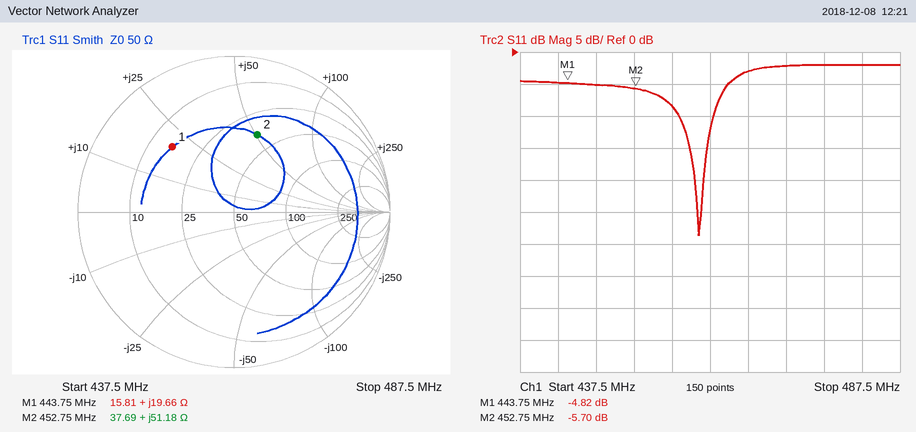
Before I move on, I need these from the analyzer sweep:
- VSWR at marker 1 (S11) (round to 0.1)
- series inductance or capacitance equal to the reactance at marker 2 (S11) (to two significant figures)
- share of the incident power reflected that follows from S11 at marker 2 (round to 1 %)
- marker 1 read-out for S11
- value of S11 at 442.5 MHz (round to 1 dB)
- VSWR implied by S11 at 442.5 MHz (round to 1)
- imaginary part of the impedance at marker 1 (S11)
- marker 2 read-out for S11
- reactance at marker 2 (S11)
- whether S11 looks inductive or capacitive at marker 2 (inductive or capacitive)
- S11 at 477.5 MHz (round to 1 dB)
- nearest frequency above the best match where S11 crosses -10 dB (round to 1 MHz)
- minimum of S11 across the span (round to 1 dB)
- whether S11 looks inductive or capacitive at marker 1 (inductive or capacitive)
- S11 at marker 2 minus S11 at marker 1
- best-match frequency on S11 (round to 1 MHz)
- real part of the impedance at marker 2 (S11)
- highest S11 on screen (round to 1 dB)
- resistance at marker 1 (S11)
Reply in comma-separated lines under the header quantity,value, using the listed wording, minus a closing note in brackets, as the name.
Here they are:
quantity,value
VSWR at marker 1 (S11),3.7
series inductance or capacitance equal to the reactance at marker 2 (S11),18 nH
share of the incident power reflected that follows from S11 at marker 2,27 %
marker 1 read-out for S11,-4.82 dB
value of S11 at 442.5 MHz,-5 dB
VSWR implied by S11 at 442.5 MHz,4
imaginary part of the impedance at marker 1,+19.66 Ω
marker 2 read-out for S11,-5.70 dB
reactance at marker 2,+51.18 Ω
whether S11 looks inductive or capacitive at marker 2,inductive
S11 at 477.5 MHz,-2 dB
nearest frequency above the best match where S11 crosses -10 dB,463 MHz
minimum of S11 across the span,-29 dB
whether S11 looks inductive or capacitive at marker 1,inductive
S11 at marker 2 minus S11 at marker 1,-0.88 dB
best-match frequency on S11,461 MHz
real part of the impedance at marker 2,37.69 Ω
highest S11 on screen,-2 dB
resistance at marker 1,15.81 Ω
